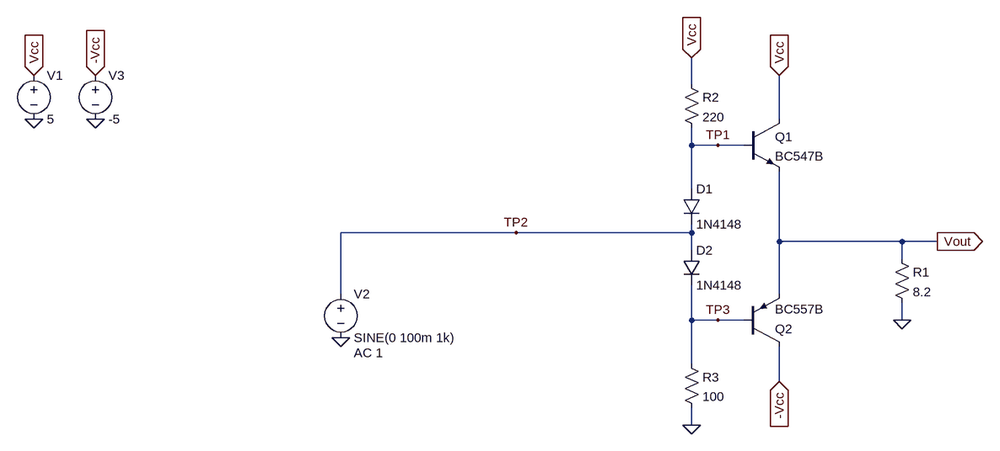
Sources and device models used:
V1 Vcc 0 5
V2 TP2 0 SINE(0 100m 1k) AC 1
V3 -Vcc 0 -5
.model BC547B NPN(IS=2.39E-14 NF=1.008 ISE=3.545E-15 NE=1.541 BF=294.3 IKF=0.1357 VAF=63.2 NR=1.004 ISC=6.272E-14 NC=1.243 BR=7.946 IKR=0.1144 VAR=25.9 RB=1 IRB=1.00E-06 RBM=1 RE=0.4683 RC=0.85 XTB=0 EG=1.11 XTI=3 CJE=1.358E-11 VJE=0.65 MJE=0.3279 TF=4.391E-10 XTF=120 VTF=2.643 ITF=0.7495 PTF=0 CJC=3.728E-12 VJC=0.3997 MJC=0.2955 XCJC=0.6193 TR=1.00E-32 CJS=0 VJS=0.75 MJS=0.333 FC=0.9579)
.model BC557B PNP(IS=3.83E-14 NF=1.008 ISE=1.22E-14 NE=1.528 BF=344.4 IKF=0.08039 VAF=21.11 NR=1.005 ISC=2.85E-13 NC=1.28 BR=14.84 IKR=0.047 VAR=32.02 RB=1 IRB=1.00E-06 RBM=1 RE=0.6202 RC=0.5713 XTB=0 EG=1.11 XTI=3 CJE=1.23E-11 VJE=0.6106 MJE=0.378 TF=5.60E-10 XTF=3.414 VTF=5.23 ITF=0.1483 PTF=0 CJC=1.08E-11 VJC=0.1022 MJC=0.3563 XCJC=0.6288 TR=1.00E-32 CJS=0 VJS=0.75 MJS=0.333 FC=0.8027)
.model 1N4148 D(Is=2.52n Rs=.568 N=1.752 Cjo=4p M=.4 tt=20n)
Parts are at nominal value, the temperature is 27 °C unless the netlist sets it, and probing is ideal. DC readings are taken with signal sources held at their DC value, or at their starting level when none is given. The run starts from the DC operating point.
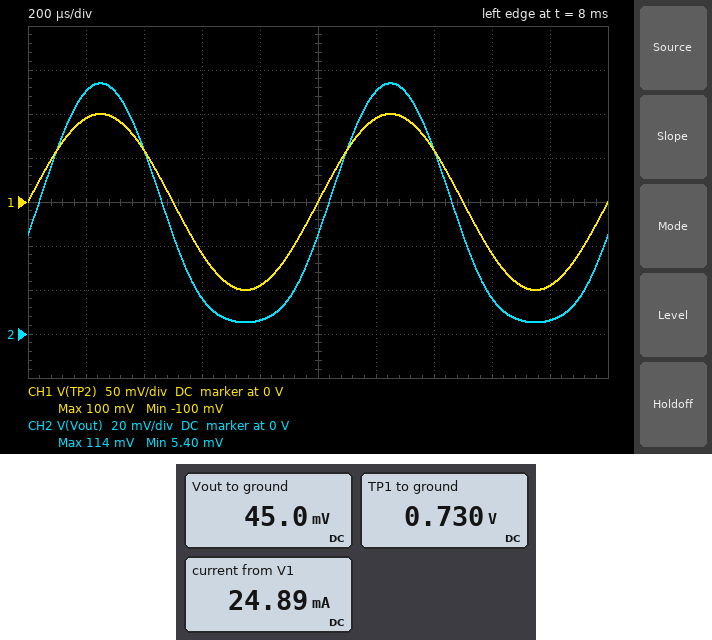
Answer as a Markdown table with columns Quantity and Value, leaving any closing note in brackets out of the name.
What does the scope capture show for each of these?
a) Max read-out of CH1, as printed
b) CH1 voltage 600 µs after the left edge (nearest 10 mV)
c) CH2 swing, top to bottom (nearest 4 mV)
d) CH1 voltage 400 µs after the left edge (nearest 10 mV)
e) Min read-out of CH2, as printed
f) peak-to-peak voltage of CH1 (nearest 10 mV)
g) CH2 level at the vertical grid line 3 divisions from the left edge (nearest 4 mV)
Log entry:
| Quantity | Value |
|---|---|
| Max read-out of CH1, as printed | 100 mV |
| CH1 voltage 600 µs after the left edge | -60 mV |
| CH2 swing, top to bottom | 108 mV |
| CH1 voltage 400 µs after the left edge | 60 mV |
| Min read-out of CH2, as printed | 5.40 mV |
| peak-to-peak voltage of CH1 | 200 mV |
| CH2 level at the vertical grid line 3 divisions from the left edge | 16 mV |
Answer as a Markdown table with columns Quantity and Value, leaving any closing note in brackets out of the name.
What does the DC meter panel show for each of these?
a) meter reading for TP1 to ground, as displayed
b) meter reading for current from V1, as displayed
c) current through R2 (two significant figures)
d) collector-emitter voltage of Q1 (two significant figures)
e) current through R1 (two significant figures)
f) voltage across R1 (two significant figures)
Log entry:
| Quantity | Value |
|---|---|
| meter reading for TP1 to ground, as displayed | 0.730 V |
| meter reading for current from V1, as displayed | 24.89 mA |
| current through R2 | 19 mA |
| collector-emitter voltage of Q1 | 5.0 V |
| current through R1 | 5.5 mA |
| voltage across R1 | 45 mV |
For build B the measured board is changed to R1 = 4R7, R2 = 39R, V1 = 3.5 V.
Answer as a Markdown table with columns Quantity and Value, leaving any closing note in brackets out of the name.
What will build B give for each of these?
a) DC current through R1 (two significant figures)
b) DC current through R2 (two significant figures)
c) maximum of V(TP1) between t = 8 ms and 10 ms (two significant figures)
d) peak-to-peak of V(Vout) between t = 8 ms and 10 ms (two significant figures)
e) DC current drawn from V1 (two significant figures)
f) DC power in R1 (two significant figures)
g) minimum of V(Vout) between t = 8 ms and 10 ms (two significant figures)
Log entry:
| Quantity | Value |
|---|---|
| DC current through R1 | 19 mA |
| DC current through R2 | 69 mA |
| maximum of V(TP1) between t = 8 ms and 10 ms | 910 mV |
| peak-to-peak of V(Vout) between t = 8 ms and 10 ms | 130 mV |
| DC current drawn from V1 | 88 mA |
| DC power in R1 | 1.7 mW |
| minimum of V(Vout) between t = 8 ms and 10 ms | 29 mV |
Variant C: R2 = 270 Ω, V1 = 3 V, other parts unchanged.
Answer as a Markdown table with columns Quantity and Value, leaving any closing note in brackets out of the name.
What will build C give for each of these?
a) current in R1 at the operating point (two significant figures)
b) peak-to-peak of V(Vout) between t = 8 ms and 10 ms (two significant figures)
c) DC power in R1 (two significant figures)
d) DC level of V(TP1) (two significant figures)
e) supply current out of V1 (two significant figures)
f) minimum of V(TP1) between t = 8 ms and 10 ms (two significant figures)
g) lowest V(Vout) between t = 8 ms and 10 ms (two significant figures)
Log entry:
| Quantity | Value |
|---|---|
| current in R1 at the operating point | 2.7 mA |
| peak-to-peak of V(Vout) between t = 8 ms and 10 ms | 79 mV |
| DC power in R1 | 58 µW |
| DC level of V(TP1) | 690 mV |
| supply current out of V1 | 11 mA |
| minimum of V(TP1) between t = 8 ms and 10 ms | 590 mV |
| lowest V(Vout) between t = 8 ms and 10 ms | 1.2 mV |
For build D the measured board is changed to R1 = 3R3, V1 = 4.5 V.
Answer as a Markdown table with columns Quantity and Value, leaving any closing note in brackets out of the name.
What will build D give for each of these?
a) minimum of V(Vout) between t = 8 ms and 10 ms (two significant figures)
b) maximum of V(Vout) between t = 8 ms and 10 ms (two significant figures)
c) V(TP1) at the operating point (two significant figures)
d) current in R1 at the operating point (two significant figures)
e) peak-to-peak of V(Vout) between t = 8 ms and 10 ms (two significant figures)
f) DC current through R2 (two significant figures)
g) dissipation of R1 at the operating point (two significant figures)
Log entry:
| Quantity | Value |
|---|---|
| minimum of V(Vout) between t = 8 ms and 10 ms | 1.9 mV |
| maximum of V(Vout) between t = 8 ms and 10 ms | 84 mV |
| V(TP1) at the operating point | 720 mV |
| current in R1 at the operating point | 8.0 mA |
| peak-to-peak of V(Vout) between t = 8 ms and 10 ms | 82 mV |
| DC current through R2 | 17 mA |
| dissipation of R1 at the operating point | 210 µW |
